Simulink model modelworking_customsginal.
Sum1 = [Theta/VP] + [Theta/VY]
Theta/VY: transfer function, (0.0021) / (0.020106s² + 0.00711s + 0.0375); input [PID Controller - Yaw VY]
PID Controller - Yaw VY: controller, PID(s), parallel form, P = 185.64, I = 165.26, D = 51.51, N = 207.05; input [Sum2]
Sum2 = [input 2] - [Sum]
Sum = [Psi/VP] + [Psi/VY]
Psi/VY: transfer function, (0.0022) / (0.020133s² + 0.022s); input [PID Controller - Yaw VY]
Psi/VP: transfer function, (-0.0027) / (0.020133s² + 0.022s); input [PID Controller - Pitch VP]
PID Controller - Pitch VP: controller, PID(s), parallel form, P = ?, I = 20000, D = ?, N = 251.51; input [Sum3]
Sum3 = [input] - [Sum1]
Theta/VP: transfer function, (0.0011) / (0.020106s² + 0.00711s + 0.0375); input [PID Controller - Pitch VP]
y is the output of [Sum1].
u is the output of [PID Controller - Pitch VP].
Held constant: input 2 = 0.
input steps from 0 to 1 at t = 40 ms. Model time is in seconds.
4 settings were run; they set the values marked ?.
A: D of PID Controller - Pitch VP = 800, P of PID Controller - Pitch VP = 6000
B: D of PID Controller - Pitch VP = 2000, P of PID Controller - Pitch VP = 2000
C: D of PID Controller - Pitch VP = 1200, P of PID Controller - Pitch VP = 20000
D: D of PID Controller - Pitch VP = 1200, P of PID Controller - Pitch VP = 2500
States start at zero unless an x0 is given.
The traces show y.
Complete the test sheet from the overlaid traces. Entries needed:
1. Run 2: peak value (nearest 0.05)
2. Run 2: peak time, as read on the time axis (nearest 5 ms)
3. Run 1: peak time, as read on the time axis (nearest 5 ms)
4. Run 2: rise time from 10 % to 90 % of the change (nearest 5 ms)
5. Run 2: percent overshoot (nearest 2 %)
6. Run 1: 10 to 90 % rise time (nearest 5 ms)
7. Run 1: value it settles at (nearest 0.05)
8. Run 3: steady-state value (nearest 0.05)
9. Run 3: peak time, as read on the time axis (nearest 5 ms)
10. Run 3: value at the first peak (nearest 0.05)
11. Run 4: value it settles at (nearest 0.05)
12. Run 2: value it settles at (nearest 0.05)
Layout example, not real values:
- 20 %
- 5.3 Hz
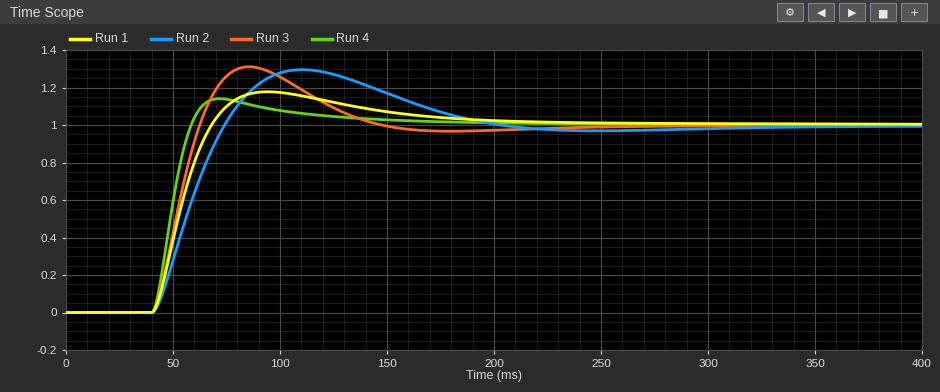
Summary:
- 1.30
- 110 ms
- 95 ms
- 25 ms
- 30 %
- 20 ms
- 1.00
- 1.00
- 85 ms
- 1.30
- 1.00
- 1.00
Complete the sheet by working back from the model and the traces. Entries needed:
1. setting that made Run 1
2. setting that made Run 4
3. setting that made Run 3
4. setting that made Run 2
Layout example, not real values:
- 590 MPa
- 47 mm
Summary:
- D
- B
- C
- A
